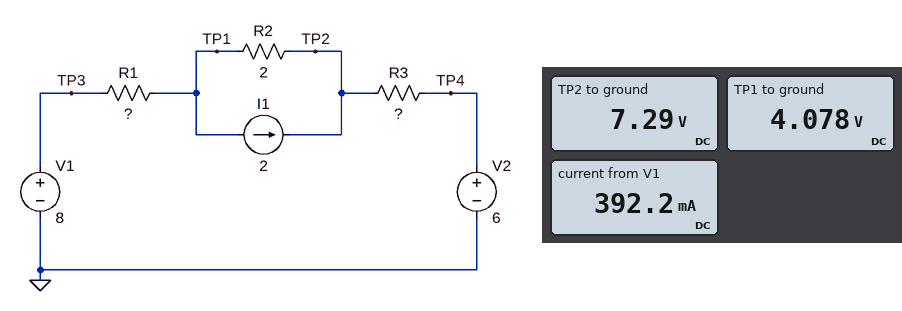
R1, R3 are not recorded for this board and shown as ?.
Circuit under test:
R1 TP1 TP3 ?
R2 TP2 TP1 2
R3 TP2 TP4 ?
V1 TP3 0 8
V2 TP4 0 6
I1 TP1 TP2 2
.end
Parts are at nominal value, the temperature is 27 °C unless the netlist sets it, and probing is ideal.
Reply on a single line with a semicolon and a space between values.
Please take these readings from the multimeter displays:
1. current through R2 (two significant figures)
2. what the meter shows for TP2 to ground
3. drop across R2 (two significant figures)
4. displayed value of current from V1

1.6 A; 7.29 V; 3.2 V; 392.2 mA
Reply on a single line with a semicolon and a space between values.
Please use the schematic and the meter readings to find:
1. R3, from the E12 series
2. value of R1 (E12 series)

3.3 Ω; 10 Ω
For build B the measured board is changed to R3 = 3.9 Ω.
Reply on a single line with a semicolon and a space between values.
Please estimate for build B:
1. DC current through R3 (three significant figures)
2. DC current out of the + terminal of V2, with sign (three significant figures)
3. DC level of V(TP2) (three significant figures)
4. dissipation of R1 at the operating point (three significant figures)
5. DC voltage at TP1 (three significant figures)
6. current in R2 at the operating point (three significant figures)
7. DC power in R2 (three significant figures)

377 mA; -377 mA; 7.47 V; 1.42 W; 4.23 V; 1.62 A; 5.27 W
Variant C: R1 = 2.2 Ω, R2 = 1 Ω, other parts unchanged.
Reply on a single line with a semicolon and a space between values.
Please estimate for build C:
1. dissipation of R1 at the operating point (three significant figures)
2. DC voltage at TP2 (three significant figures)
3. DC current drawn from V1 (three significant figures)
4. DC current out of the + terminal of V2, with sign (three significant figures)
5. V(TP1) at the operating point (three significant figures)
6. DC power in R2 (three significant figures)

833 mW; 8.03 V; 615 mA; -615 mA; 6.65 V; 1.92 W
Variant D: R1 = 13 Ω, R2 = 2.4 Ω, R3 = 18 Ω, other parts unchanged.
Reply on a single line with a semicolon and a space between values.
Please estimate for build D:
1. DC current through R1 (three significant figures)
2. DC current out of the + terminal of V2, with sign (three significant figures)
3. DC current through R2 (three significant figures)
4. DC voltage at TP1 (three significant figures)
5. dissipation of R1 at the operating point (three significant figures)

204 mA; -204 mA; 1.80 A; 5.35 V; 539 mW
